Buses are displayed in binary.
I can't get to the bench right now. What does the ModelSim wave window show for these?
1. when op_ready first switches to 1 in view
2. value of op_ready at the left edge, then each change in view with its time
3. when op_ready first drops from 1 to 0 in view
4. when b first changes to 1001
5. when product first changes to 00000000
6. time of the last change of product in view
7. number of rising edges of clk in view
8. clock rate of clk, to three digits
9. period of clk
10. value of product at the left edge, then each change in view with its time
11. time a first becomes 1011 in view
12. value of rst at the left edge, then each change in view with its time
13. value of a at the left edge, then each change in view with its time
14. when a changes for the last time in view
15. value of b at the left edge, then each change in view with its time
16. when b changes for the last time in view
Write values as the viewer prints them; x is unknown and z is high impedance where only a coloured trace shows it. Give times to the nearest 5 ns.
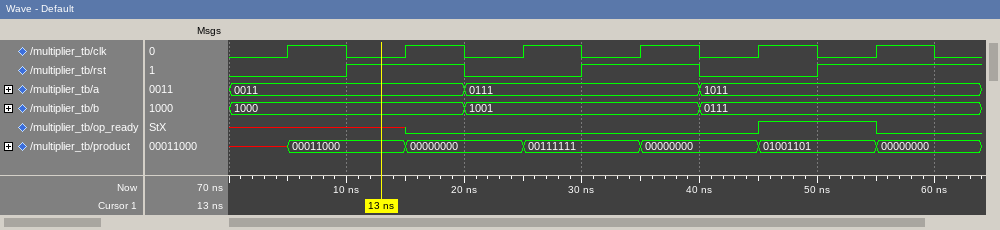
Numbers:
45 ns
x, 0 at 15 ns, 1 at 45 ns, 0 at 55 ns
55 ns
20 ns
15 ns
55 ns
6
100 MHz
10 ns
x, 00011000 at 5 ns, 00000000 at 15 ns, 00111111 at 25 ns, 00000000 at 35 ns, 01001101 at 45 ns, 00000000 at 55 ns
40 ns
0, 1 at 10 ns, 0 at 20 ns, 1 at 30 ns, 0 at 40 ns, 1 at 50 ns
0011, 0111 at 20 ns, 1011 at 40 ns
40 ns
1000, 1001 at 20 ns, 0111 at 40 ns
40 ns
